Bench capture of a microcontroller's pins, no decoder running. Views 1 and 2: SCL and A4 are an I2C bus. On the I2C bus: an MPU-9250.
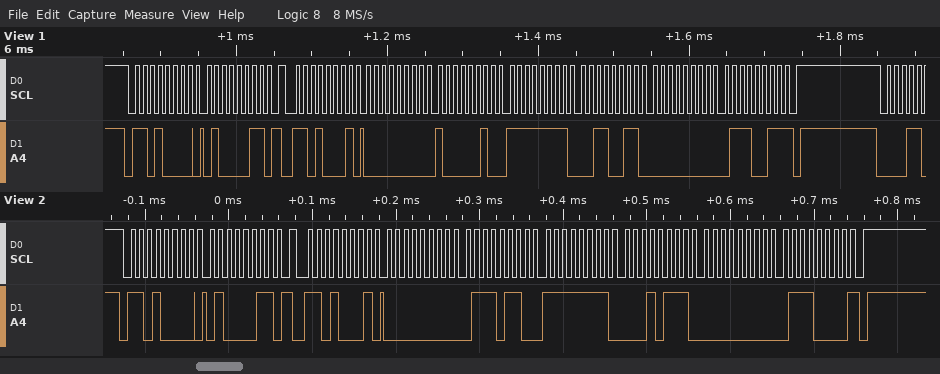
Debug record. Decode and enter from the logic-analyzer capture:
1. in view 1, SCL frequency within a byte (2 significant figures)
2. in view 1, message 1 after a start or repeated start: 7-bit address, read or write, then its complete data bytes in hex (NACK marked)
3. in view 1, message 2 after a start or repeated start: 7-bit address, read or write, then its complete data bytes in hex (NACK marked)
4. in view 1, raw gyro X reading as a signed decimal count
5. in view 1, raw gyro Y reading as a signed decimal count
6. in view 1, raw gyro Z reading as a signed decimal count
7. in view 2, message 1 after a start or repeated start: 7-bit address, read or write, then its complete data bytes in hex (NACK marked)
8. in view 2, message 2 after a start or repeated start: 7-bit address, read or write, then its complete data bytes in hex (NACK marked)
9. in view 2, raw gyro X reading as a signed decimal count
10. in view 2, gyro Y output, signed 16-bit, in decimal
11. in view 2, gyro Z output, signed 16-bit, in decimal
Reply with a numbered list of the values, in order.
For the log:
1. 100 kHz
2. 0x68 write: 43
3. 0x68 read: 00 82 FF 33 00 73 NACK
4. 130
5. -205
6. 115
7. 0x68 write: 43
8. 0x68 read: 00 76 FF 17 00 70 NACK
9. 118
10. -233
11. 112
